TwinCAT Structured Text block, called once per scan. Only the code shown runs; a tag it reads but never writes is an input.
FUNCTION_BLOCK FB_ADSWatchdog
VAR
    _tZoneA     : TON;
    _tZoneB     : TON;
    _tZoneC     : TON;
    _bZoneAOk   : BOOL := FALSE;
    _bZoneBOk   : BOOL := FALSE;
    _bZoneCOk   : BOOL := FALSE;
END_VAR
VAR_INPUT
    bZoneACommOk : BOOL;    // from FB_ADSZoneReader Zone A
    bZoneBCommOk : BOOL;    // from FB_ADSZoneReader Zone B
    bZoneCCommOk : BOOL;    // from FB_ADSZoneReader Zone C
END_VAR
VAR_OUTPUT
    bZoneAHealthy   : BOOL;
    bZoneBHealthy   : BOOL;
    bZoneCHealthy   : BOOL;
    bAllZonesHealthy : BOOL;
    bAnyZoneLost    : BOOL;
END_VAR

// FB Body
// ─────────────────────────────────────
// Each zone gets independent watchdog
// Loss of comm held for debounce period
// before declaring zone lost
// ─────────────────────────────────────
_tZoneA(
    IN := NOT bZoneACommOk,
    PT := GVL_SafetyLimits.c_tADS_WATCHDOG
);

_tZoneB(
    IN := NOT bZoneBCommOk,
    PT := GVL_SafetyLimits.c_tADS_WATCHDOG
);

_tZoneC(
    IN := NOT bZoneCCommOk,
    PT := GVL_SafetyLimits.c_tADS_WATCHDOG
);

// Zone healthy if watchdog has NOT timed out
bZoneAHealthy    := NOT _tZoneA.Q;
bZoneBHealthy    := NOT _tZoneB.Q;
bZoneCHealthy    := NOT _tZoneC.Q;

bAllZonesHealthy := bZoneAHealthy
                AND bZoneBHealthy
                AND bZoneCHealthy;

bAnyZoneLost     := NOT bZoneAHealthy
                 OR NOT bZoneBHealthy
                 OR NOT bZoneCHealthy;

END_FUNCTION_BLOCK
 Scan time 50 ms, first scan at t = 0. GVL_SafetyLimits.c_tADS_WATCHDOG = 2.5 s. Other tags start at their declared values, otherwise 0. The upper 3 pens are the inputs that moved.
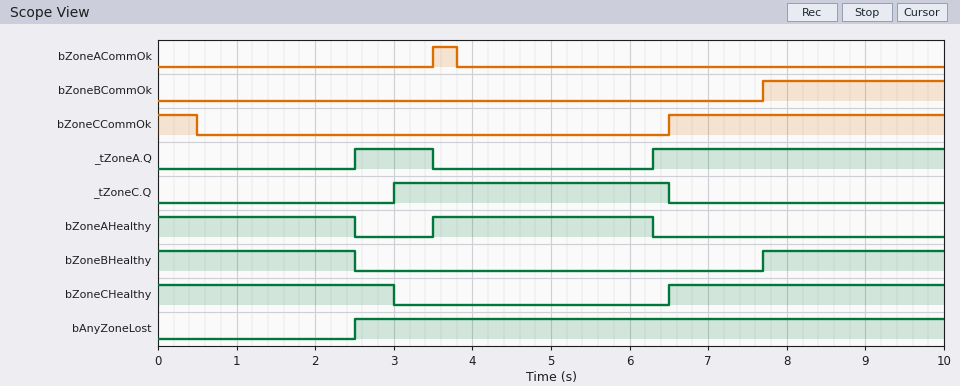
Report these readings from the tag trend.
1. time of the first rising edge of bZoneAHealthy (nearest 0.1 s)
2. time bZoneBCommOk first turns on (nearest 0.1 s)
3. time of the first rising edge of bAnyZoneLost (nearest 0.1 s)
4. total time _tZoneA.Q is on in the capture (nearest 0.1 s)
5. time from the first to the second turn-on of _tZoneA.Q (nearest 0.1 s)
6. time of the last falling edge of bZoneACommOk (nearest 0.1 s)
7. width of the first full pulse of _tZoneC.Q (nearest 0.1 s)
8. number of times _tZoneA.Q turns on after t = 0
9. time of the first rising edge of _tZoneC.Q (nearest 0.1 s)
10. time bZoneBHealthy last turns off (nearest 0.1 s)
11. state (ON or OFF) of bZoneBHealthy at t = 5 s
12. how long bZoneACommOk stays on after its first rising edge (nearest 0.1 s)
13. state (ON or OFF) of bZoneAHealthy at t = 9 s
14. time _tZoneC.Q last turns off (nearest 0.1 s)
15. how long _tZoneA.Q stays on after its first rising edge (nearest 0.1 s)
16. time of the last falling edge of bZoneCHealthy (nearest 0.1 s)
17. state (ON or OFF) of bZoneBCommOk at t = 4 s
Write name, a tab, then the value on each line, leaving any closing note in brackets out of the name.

time of the first rising edge of bZoneAHealthy	3.5 s
time bZoneBCommOk first turns on	7.7 s
time of the first rising edge of bAnyZoneLost	2.5 s
total time _tZoneA.Q is on in the capture	4.7 s
time from the first to the second turn-on of _tZoneA.Q	3.8 s
time of the last falling edge of bZoneACommOk	3.8 s
width of the first full pulse of _tZoneC.Q	3.5 s
number of times _tZoneA.Q turns on after t = 0	2
time of the first rising edge of _tZoneC.Q	3.0 s
time bZoneBHealthy last turns off	2.5 s
state (ON or OFF) of bZoneBHealthy at t = 5 s	OFF
how long bZoneACommOk stays on after its first rising edge	0.3 s
state (ON or OFF) of bZoneAHealthy at t = 9 s	OFF
time _tZoneC.Q last turns off	6.5 s
how long _tZoneA.Q stays on after its first rising edge	1.0 s
time of the last falling edge of bZoneCHealthy	3.0 s
state (ON or OFF) of bZoneBCommOk at t = 4 s	OFF
